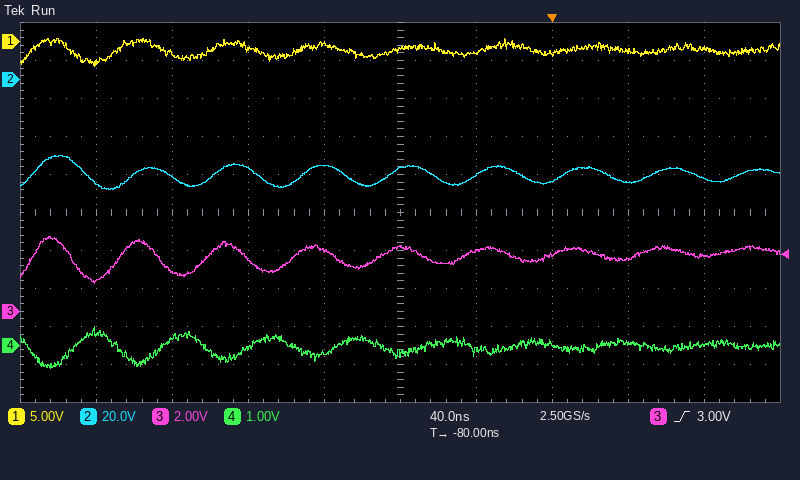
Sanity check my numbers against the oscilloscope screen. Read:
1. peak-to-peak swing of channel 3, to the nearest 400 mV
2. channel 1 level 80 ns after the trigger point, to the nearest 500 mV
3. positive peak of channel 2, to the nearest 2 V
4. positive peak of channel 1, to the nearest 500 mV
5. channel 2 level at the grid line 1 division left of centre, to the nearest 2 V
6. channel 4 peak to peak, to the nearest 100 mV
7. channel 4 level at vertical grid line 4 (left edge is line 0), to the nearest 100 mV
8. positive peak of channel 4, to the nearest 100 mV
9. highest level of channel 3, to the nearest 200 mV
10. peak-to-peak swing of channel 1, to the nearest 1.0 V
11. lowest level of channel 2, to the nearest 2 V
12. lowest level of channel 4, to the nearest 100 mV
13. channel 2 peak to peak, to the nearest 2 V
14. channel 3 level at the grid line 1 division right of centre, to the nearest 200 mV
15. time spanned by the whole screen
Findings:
2.4 V
-1.0 V
-40 V
500 mV
-46 V
1.1 V
-200 mV
500 mV
4.0 V
4.0 V
-58 V
-600 mV
18 V
3.2 V
400 ns
